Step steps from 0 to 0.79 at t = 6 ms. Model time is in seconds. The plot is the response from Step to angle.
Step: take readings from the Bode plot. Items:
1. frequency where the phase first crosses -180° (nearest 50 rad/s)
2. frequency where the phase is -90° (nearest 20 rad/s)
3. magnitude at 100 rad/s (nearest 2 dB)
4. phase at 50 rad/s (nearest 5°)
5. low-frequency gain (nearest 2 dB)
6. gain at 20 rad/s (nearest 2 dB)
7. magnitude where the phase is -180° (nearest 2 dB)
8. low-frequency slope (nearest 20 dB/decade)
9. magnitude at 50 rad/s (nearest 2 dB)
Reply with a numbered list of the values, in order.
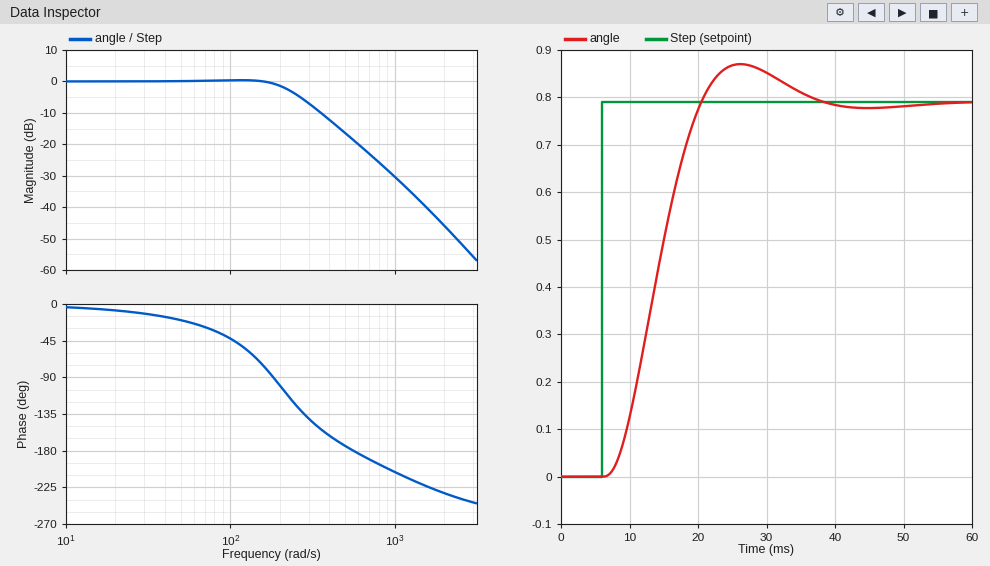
1. 550 rad/s
2. 180 rad/s
3. 0 dB
4. -20°
5. 0 dB
6. 0 dB
7. -18 dB
8. 0 dB/decade
9. 0 dB
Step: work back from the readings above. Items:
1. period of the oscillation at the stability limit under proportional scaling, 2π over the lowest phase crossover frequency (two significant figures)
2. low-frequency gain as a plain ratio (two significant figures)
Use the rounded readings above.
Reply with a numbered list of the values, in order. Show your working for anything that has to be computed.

1. 2π / 550 = 0.011 s
2. 10^(0 / 20) = 1.0
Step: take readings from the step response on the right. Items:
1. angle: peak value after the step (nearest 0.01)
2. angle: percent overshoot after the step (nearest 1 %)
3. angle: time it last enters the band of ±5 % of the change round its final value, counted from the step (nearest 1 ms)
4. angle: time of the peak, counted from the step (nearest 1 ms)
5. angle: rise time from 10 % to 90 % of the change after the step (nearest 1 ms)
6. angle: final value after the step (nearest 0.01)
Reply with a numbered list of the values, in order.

1. 0.87
2. 10 %
3. 27 ms
4. 20 ms
5. 9 ms
6. 0.79
